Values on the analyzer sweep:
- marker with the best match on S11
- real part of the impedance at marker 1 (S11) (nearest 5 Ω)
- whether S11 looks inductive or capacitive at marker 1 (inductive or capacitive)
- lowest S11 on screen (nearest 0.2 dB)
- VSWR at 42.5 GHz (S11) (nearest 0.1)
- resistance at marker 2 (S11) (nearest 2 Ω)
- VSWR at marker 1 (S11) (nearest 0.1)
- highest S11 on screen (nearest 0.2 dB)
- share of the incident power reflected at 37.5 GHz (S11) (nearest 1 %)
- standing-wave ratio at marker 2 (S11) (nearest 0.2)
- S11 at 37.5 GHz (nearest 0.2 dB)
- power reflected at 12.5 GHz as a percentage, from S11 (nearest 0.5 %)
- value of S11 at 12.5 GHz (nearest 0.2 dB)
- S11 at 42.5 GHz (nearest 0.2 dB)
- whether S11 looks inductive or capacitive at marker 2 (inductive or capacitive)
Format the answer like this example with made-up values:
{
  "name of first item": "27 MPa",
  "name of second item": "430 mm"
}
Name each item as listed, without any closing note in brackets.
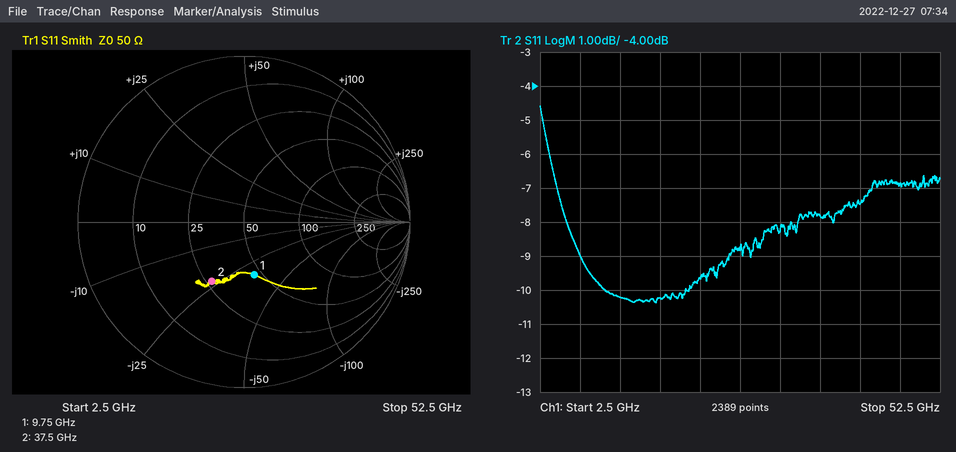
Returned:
{
  "marker with the best match on S11": "marker 1",
  "real part of the impedance at marker 1 (S11)": "45 Ω",
  "whether S11 looks inductive or capacitive at marker 1": "capacitive",
  "lowest S11 on screen": "-10.4 dB",
  "VSWR at 42.5 GHz (S11)": "2.5",
  "resistance at marker 2 (S11)": "26 Ω",
  "VSWR at marker 1 (S11)": "2.0",
  "highest S11 on screen": "-4.6 dB",
  "share of the incident power reflected at 37.5 GHz (S11)": "17 %",
  "standing-wave ratio at marker 2 (S11)": "2.4",
  "S11 at 37.5 GHz": "-7.8 dB",
  "power reflected at 12.5 GHz as a percentage, from S11": "9.5 %",
  "value of S11 at 12.5 GHz": "-10.2 dB",
  "S11 at 42.5 GHz": "-7.4 dB",
  "whether S11 looks inductive or capacitive at marker 2": "capacitive"
}
